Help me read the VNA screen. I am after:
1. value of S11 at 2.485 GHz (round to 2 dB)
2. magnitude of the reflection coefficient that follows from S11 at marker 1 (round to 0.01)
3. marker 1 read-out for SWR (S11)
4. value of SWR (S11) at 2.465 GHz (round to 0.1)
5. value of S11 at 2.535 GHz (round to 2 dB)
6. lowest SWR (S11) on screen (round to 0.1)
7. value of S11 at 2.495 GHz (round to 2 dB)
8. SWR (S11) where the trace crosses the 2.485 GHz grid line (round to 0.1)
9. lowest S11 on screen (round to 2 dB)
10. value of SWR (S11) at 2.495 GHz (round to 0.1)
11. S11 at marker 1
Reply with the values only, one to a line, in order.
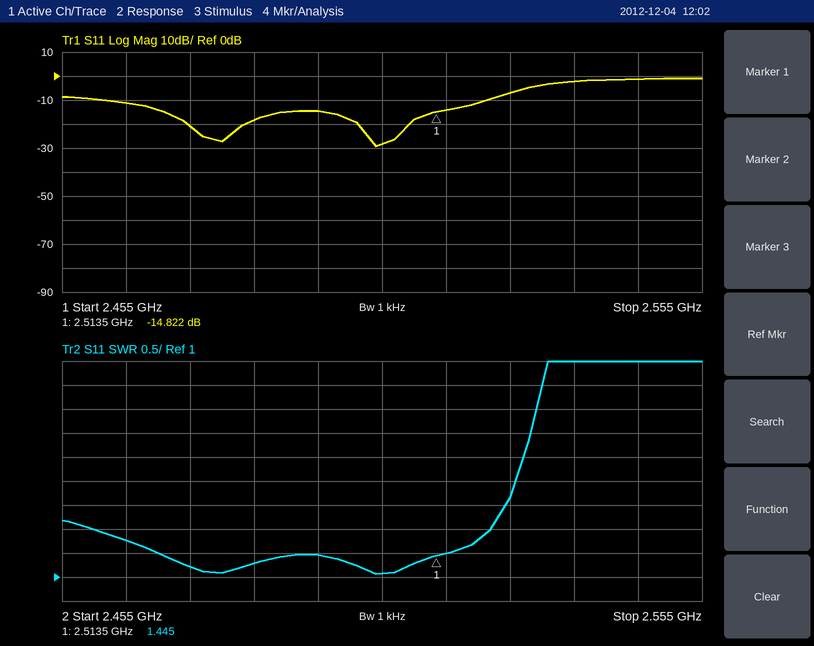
-18 dB
0.18
1.445
1.8
-2 dB
1.1
-14 dB
1.3
-30 dB
1.5
-14.822 dB
